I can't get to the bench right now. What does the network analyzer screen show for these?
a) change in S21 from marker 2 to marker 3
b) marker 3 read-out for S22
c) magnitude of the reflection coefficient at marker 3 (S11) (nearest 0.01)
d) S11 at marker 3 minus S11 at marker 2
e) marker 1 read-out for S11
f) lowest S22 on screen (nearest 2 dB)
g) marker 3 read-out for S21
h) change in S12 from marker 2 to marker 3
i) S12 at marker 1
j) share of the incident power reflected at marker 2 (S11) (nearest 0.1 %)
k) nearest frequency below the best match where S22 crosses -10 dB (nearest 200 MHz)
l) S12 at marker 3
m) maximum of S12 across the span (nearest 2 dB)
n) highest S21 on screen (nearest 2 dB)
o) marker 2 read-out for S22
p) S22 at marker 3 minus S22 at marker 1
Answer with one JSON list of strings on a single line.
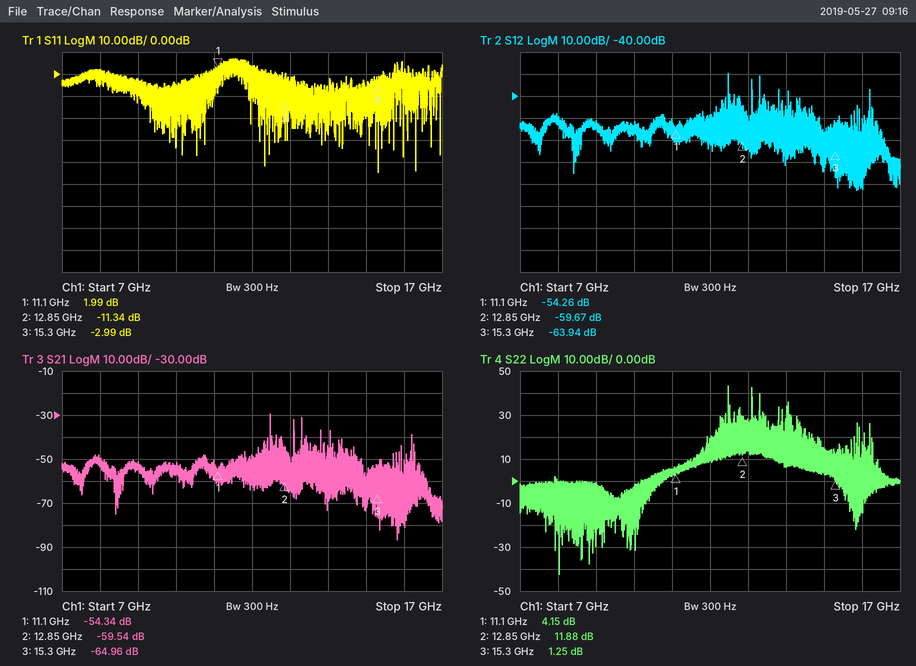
["-5.42 dB", "1.25 dB", "0.71", "8.35 dB", "1.99 dB", "-42 dB", "-64.96 dB", "-4.27 dB", "-54.26 dB", "7.3 %", "8.0 GHz", "-63.94 dB", "-30 dB", "-30 dB", "11.88 dB", "-2.90 dB"]
